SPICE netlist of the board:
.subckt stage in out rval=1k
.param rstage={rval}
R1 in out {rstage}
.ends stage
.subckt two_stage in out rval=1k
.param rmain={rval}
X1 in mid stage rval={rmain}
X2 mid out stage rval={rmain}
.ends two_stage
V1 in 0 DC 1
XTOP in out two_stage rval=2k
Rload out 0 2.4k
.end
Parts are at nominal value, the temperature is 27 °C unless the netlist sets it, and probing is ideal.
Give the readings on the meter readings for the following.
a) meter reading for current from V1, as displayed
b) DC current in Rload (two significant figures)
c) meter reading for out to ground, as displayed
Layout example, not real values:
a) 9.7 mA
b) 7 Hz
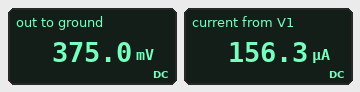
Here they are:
a) 156.3 µA
b) 160 µA
c) 375.0 mV
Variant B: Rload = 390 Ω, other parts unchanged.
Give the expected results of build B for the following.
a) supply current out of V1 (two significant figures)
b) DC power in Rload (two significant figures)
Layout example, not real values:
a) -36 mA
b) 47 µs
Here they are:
a) 230 µA
b) 20 µW
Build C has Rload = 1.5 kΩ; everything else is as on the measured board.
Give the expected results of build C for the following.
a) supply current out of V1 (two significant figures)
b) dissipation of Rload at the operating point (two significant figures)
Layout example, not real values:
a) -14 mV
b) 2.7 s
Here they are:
a) 180 µA
b) 50 µW
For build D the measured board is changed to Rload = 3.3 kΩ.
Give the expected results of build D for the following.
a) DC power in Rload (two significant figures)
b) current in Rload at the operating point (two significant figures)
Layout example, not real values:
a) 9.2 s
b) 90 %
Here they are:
a) 62 µW
b) 140 µA
